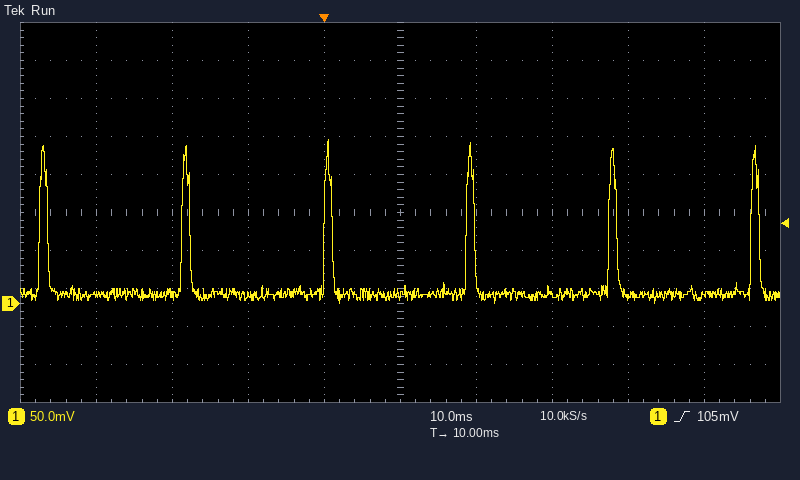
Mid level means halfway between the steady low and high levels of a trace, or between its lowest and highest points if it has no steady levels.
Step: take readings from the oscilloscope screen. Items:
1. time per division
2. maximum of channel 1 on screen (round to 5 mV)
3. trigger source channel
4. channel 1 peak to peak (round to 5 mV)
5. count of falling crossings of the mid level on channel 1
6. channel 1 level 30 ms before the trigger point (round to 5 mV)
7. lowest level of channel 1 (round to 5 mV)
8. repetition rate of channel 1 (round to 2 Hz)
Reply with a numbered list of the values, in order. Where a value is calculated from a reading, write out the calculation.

1. 10 ms
2. 215 mV
3. channel 1
4. 215 mV − (0 mV) = 215 mV
5. 6
6. 10 mV
7. 0 mV
8. 54 Hz
